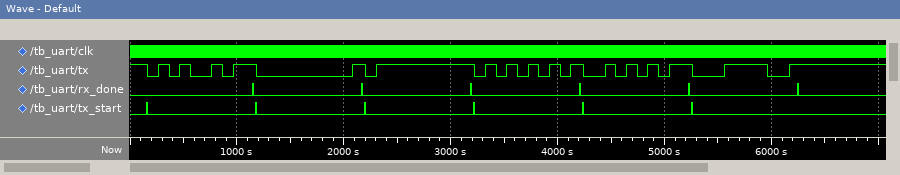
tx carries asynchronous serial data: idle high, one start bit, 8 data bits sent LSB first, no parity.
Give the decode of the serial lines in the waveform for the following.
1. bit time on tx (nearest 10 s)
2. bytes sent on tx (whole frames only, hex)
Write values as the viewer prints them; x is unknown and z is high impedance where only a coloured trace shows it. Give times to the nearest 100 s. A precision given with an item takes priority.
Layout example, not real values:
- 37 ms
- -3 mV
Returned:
- 100 s
- A5, 00, FF, 55, AA, 3C
